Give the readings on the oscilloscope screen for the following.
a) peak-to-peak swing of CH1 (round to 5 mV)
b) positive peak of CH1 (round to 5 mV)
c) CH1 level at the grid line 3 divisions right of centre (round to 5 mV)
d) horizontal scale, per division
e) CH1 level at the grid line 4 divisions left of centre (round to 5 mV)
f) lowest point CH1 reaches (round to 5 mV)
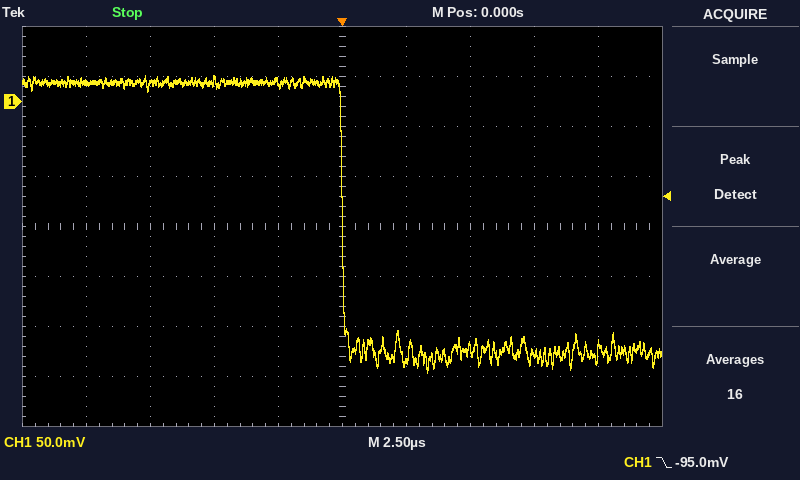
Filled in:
295 mV
25 mV
-250 mV
2.5 µs
20 mV
-270 mV
